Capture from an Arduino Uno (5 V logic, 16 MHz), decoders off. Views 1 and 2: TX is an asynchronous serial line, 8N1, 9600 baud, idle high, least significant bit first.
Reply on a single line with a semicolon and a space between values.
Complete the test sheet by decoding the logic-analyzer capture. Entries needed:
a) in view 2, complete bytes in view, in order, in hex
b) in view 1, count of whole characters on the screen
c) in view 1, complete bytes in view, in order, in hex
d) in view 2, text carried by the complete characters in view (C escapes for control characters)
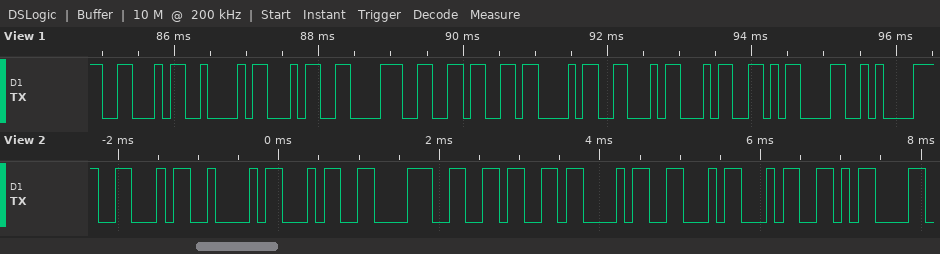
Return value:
46 42 34 38 36 43 46 34 0D; 10; 46 42 34 38 36 43 46 34 0D 0A; "FB486CF4\r"
